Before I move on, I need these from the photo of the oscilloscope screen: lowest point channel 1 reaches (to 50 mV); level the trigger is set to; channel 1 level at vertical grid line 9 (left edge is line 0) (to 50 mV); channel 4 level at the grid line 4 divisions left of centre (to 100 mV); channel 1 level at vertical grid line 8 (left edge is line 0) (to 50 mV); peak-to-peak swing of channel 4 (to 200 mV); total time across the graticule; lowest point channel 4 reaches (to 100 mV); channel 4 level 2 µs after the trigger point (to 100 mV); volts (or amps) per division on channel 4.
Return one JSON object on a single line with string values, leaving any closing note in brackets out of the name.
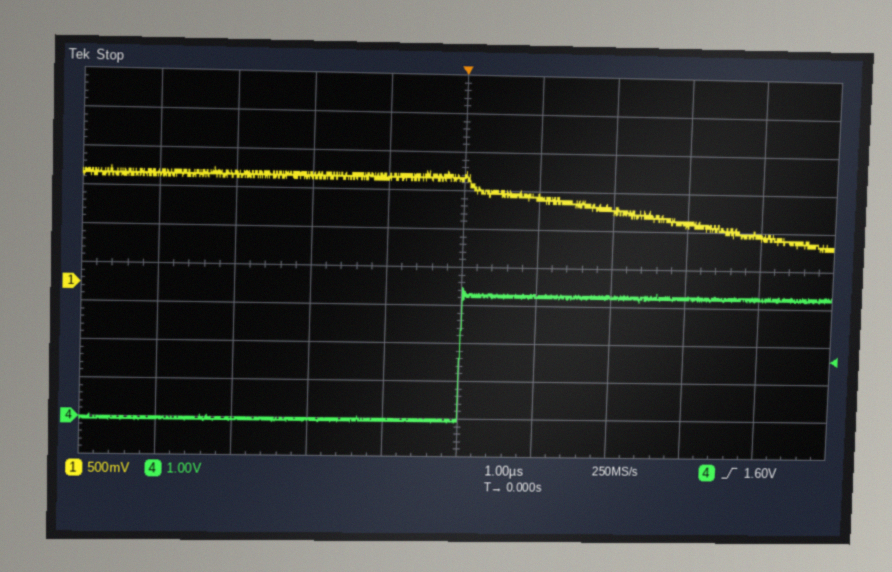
{"lowest point channel 1 reaches": "550 mV", "level the trigger is set to": "1.60 V", "channel 1 level at vertical grid line 9 (left edge is line 0)": "700 mV", "channel 4 level at the grid line 4 divisions left of centre": "0.0 V", "channel 1 level at vertical grid line 8 (left edge is line 0)": "850 mV", "peak-to-peak swing of channel 4": "3.6 V", "total time across the graticule": "10 µs", "lowest point channel 4 reaches": "-100 mV", "channel 4 level 2 µs after the trigger point": "3.3 V", "volts (or amps) per division on channel 4": "1 V"}
